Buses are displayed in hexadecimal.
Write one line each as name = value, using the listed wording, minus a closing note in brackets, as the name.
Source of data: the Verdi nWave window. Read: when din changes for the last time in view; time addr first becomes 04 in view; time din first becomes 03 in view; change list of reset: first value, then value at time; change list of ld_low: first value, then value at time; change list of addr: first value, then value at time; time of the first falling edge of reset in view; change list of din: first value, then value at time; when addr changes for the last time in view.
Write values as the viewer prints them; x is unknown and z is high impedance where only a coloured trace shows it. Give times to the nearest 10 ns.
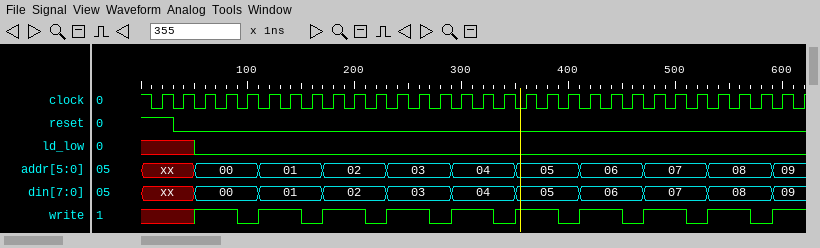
when din changes for the last time in view = 590 ns
time addr first becomes 04 in view = 290 ns
time din first becomes 03 in view = 230 ns
change list of reset: first value, then value at time = 1, 0 at 30 ns
change list of ld_low: first value, then value at time = x, 0 at 50 ns
change list of addr: first value, then value at time = xx, 00 at 50 ns, 01 at 110 ns, 02 at 170 ns, 03 at 230 ns, 04 at 290 ns, 05 at 350 ns, 06 at 410 ns, 07 at 470 ns, 08 at 530 ns, 09 at 590 ns
time of the first falling edge of reset in view = 30 ns
change list of din: first value, then value at time = xx, 00 at 50 ns, 01 at 110 ns, 02 at 170 ns, 03 at 230 ns, 04 at 290 ns, 05 at 350 ns, 06 at 410 ns, 07 at 470 ns, 08 at 530 ns, 09 at 590 ns
when addr changes for the last time in view = 590 ns
